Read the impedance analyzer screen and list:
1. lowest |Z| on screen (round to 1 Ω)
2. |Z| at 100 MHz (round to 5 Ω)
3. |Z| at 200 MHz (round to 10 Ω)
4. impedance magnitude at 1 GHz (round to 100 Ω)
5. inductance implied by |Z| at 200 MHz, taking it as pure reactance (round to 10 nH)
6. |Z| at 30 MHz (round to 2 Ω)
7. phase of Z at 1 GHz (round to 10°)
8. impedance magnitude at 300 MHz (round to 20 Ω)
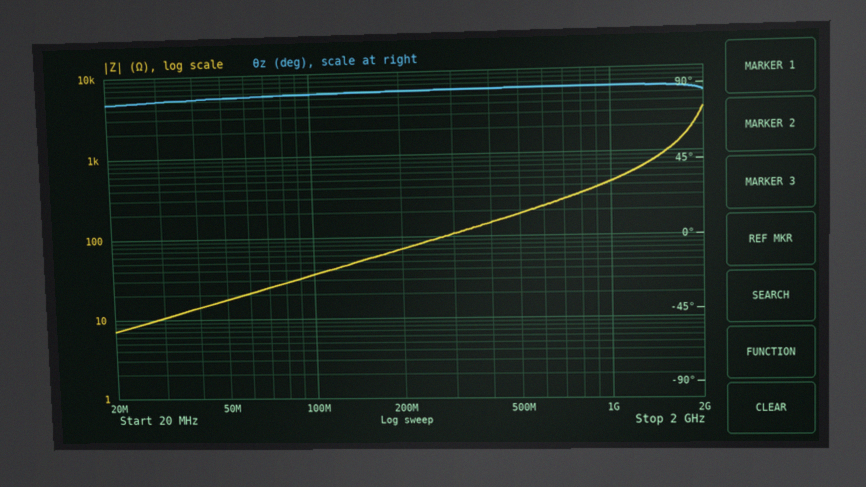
7 Ω
35 Ω
70 Ω
400 Ω
60 nH
10 Ω
90°
100 Ω
